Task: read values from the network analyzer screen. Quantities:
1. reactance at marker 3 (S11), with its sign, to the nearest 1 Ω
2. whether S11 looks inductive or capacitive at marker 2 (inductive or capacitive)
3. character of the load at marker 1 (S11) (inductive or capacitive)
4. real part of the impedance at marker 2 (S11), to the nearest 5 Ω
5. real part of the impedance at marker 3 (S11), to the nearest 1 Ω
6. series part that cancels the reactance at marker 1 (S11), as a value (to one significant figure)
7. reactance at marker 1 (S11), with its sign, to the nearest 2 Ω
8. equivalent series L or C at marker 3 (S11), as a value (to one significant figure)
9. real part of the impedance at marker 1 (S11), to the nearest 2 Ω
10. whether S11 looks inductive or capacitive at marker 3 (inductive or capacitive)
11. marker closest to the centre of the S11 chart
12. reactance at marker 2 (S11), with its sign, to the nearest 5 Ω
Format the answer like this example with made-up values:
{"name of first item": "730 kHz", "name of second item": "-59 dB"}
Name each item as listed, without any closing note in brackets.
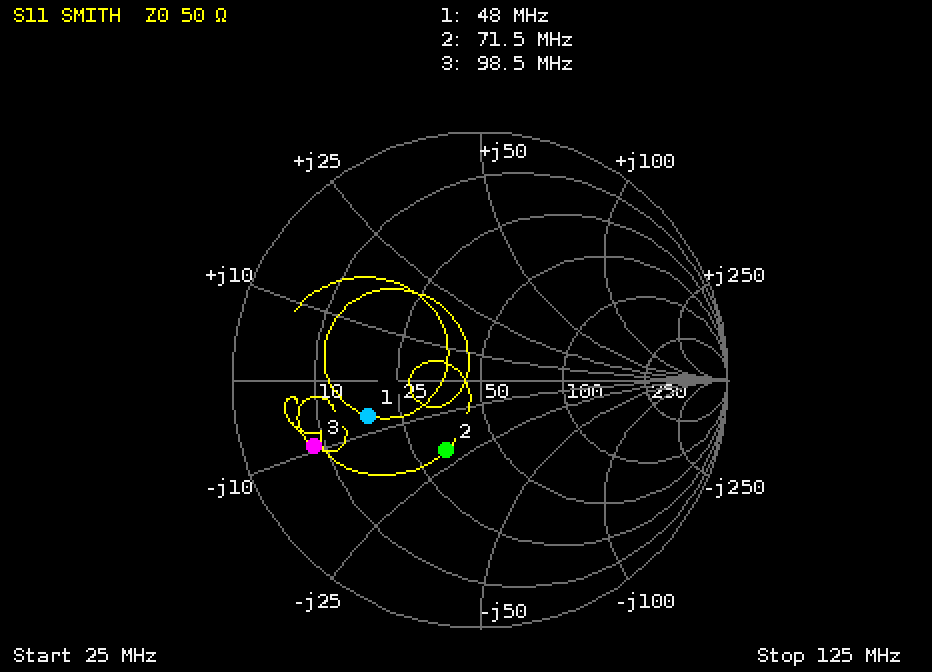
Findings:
{"reactance at marker 3 (S11), with its sign, to the nearest 1 Ω": "-9 Ω", "whether S11 looks inductive or capacitive at marker 2": "capacitive", "character of the load at marker 1 (S11)": "capacitive", "real part of the impedance at marker 2 (S11), to the nearest 5 Ω": "35 Ω", "real part of the impedance at marker 3 (S11), to the nearest 1 Ω": "8 Ω", "series part that cancels the reactance at marker 1 (S11), as a value": "20 nH", "reactance at marker 1 (S11), with its sign, to the nearest 2 Ω": "-6 Ω", "equivalent series L or C at marker 3 (S11), as a value": "200 pF", "real part of the impedance at marker 1 (S11), to the nearest 2 Ω": "18 Ω", "whether S11 looks inductive or capacitive at marker 3": "capacitive", "marker closest to the centre of the S11 chart": "marker 2", "reactance at marker 2 (S11), with its sign, to the nearest 5 Ω": "-20 Ω"}
